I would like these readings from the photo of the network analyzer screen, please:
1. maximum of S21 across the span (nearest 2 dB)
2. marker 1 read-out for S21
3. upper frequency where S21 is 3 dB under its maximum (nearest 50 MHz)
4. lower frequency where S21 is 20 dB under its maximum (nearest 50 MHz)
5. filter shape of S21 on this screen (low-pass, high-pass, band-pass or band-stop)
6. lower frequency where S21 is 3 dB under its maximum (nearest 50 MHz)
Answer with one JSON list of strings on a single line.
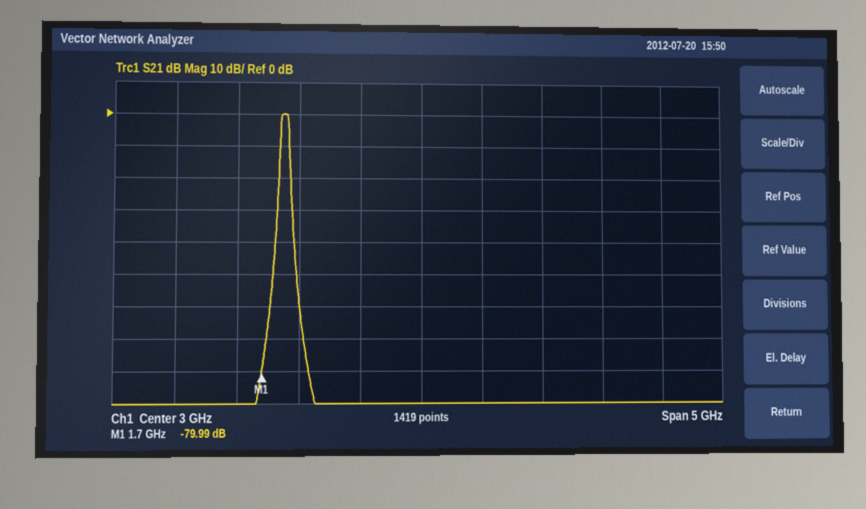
["0 dB", "-79.99 dB", "1.90 GHz", "1.85 GHz", "band-pass", "1.85 GHz"]
